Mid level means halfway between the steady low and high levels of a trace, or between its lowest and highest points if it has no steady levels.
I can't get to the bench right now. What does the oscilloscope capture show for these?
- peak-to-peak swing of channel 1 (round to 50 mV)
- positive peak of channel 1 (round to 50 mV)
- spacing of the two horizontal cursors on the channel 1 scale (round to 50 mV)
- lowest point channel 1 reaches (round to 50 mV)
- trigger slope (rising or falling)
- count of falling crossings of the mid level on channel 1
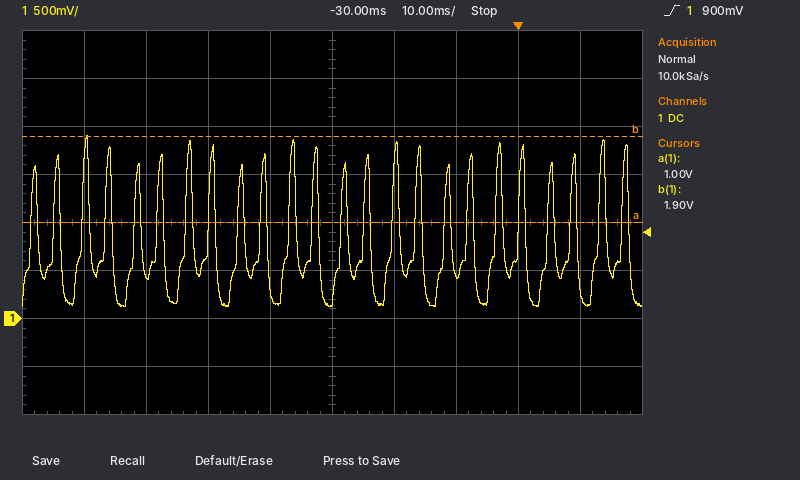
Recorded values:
1.80 V
1.90 V
900 mV
100 mV
rising
24
